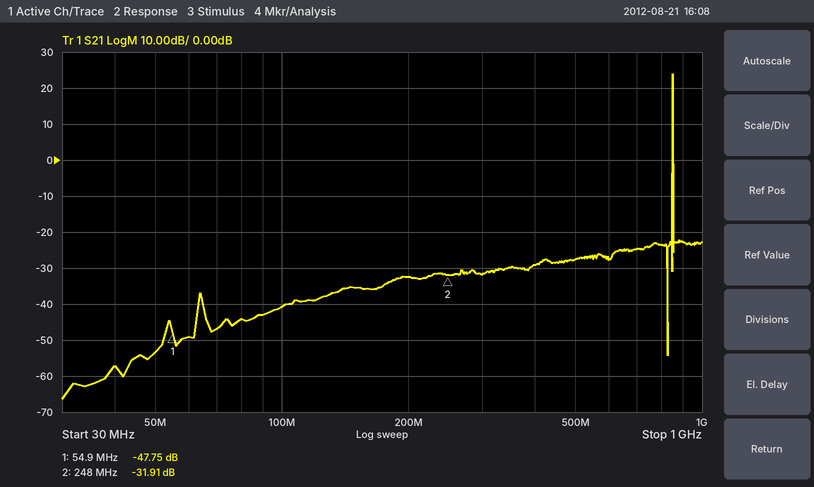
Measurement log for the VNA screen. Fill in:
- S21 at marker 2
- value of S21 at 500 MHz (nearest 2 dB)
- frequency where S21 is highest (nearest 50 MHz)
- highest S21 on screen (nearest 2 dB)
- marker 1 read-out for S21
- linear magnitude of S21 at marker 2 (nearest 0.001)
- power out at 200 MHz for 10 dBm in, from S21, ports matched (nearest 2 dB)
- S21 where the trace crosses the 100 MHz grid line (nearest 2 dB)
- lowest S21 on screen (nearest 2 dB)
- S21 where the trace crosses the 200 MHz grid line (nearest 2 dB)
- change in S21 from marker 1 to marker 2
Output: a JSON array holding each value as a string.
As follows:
["-31.91 dB", "-28 dB", "850 MHz", "24 dB", "-47.75 dB", "0.025", "-22 dBm", "-40 dB", "-66 dB", "-32 dB", "15.84 dB"]
